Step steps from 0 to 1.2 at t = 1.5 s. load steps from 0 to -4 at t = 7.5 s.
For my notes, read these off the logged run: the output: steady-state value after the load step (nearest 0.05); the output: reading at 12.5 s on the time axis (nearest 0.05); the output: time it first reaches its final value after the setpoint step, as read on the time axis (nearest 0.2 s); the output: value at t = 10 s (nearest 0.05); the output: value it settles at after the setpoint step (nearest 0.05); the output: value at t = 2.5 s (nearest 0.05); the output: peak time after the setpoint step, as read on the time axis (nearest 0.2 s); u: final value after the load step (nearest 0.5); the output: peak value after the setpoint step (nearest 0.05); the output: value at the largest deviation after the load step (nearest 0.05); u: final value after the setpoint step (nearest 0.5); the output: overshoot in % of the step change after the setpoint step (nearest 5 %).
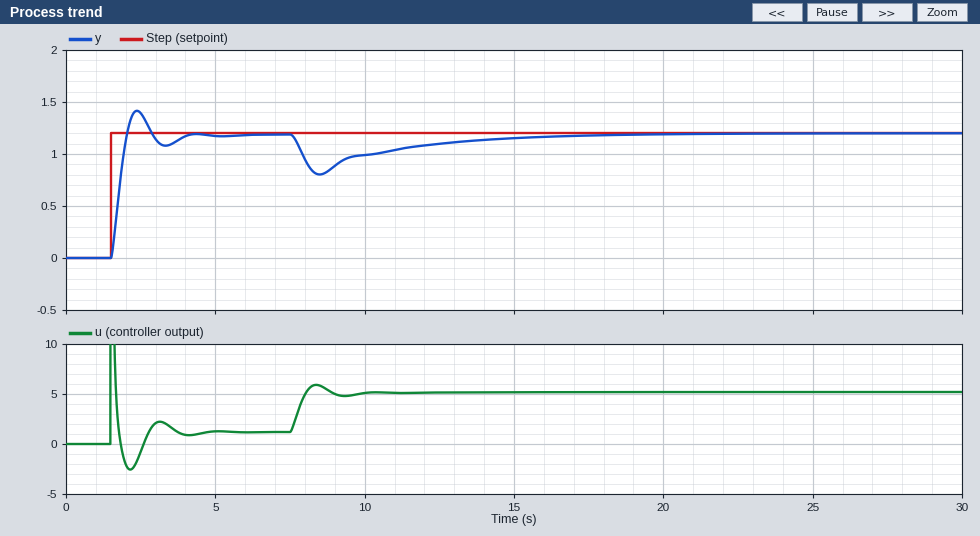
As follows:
1.20
1.10
2.0 s
1.00
1.20
1.40
2.4 s
5.0
1.40
0.80
1.0
20 %
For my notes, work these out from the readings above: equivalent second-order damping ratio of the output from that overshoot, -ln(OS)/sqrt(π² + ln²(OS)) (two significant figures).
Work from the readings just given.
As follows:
0.46
